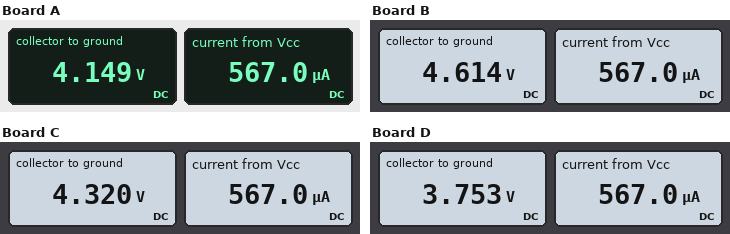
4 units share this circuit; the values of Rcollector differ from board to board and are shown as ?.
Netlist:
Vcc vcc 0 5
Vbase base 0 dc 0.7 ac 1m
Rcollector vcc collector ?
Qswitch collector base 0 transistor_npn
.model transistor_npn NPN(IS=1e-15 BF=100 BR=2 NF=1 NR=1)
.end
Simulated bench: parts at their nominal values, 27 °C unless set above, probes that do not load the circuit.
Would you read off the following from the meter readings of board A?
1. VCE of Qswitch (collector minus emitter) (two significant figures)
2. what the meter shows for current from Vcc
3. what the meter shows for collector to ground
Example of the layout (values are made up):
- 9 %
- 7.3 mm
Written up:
- 4.1 V
- 567.0 µA
- 4.149 V
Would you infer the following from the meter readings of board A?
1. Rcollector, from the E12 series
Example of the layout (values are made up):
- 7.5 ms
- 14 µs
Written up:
- 1.5 kΩ
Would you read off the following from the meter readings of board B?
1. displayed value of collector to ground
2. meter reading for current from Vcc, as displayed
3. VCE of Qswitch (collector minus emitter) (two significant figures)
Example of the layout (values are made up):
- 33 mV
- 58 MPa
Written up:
- 4.614 V
- 567.0 µA
- 4.6 V
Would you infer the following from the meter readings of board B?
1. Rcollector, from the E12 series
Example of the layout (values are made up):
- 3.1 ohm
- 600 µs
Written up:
- 680 Ω
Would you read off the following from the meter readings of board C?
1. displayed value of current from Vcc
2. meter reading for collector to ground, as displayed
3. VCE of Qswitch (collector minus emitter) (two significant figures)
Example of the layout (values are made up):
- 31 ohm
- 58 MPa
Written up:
- 567.0 µA
- 4.320 V
- 4.3 V
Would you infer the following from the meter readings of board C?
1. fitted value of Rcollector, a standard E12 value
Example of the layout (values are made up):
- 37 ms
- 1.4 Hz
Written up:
- 1.2 kΩ
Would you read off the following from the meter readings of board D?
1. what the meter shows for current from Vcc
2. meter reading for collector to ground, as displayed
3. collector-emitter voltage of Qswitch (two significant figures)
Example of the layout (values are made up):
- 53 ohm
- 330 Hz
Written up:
- 567.0 µA
- 3.753 V
- 3.8 V
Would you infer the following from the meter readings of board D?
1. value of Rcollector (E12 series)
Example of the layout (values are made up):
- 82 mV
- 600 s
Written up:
- 2.2 kΩ
